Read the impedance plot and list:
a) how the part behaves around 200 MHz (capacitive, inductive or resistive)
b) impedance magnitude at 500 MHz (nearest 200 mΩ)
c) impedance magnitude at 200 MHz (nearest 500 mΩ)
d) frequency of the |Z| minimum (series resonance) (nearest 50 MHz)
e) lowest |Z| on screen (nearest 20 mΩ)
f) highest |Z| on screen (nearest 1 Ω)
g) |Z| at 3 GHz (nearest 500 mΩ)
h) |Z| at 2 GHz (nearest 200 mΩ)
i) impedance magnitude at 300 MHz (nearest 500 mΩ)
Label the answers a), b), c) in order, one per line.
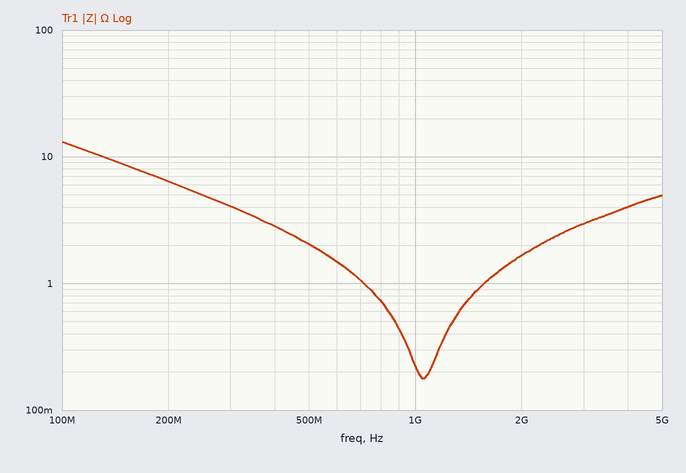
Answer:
a) capacitive
b) 2.0 Ω
c) 6.5 Ω
d) 1.05 GHz
e) 180 mΩ
f) 13 Ω
g) 3.0 Ω
h) 1.6 Ω
i) 4.0 Ω
